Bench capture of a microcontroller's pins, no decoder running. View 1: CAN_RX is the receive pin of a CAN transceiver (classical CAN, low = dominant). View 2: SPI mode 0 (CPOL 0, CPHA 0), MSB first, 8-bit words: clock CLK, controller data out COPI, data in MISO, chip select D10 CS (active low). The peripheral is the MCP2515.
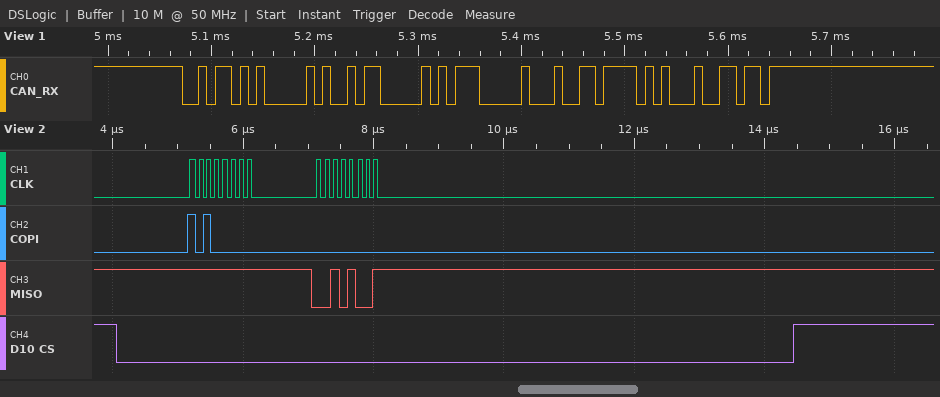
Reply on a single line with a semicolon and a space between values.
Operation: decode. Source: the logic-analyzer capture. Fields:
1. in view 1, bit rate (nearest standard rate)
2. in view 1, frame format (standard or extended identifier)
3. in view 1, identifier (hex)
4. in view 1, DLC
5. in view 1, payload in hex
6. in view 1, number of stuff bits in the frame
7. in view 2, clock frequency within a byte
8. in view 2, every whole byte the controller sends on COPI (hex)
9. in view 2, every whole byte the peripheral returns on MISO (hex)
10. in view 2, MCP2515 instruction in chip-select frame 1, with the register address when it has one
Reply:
125 kbit/s; standard; 0x2D4; 4; B0 2E 01 37; 3; 8 MHz; 0xA0 0x00; 0xFF 0x29; READ STATUS
